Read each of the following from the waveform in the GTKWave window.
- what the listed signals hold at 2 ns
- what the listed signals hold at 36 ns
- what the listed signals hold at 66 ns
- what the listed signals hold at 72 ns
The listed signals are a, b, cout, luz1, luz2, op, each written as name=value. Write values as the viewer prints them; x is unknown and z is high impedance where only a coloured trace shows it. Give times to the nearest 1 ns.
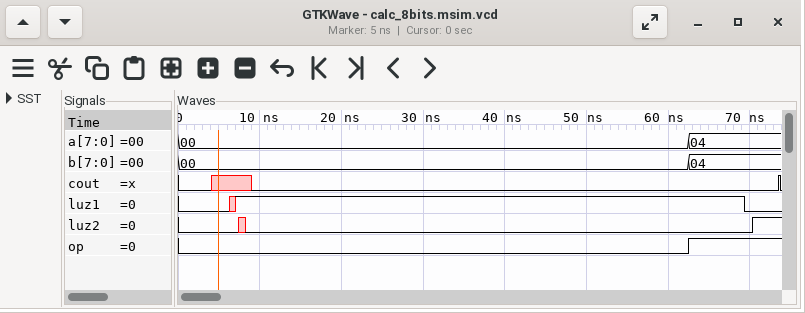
a=00, b=00, cout=0, luz1=0, luz2=0, op=0
a=00, b=00, cout=0, luz1=1, luz2=0, op=0
a=04, b=04, cout=0, luz1=1, luz2=0, op=1
a=04, b=04, cout=0, luz1=0, luz2=1, op=1
